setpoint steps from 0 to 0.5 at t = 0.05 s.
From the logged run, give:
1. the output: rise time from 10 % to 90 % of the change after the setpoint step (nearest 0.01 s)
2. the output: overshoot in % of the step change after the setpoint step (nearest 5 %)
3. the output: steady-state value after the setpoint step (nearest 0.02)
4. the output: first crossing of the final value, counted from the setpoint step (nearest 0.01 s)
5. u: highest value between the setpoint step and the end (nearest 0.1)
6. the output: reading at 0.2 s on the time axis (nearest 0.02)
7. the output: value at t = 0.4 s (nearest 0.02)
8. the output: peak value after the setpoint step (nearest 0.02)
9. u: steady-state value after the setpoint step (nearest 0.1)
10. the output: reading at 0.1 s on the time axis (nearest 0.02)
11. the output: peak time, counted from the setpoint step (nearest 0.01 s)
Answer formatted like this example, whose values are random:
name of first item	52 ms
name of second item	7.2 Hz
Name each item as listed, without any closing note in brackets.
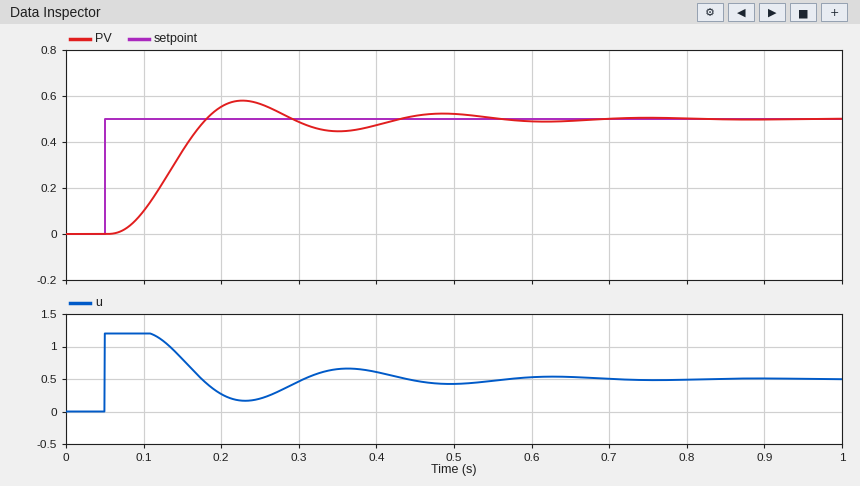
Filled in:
the output: rise time from 10 % to 90 % of the change after the setpoint step	0.08 s
the output: overshoot in % of the step change after the setpoint step	15 %
the output: steady-state value after the setpoint step	0.50
the output: first crossing of the final value, counted from the setpoint step	0.13 s
u: highest value between the setpoint step and the end	1.2
the output: reading at 0.2 s on the time axis	0.56
the output: value at t = 0.4 s	0.48
the output: peak value after the setpoint step	0.58
u: steady-state value after the setpoint step	0.5
the output: reading at 0.1 s on the time axis	0.10
the output: peak time, counted from the setpoint step	0.18 s
